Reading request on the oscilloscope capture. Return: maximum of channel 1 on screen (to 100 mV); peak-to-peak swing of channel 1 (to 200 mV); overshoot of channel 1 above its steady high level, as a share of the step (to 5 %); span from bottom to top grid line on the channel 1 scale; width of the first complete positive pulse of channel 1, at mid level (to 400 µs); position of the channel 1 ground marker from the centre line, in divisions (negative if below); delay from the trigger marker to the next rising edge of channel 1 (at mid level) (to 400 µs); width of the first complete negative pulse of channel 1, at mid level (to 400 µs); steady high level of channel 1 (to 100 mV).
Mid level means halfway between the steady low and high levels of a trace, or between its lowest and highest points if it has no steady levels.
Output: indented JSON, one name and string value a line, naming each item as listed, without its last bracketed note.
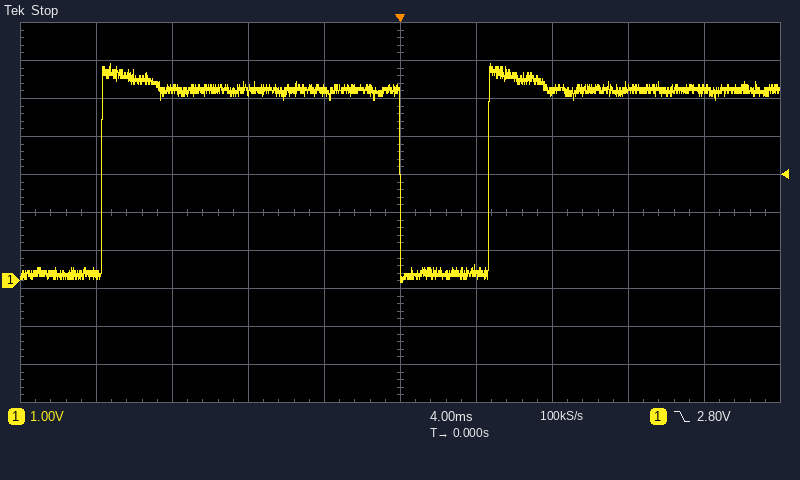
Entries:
{
  "maximum of channel 1 on screen": "5.7 V",
  "peak-to-peak swing of channel 1": "5.8 V",
  "overshoot of channel 1 above its steady high level, as a share of the step": "15 %",
  "span from bottom to top grid line on the channel 1 scale": "10 V",
  "width of the first complete positive pulse of channel 1, at mid level": "15.6 ms",
  "position of the channel 1 ground marker from the centre line, in divisions": "-1.8 div",
  "delay from the trigger marker to the next rising edge of channel 1 (at mid level)": "4.8 ms",
  "width of the first complete negative pulse of channel 1, at mid level": "4.8 ms",
  "steady high level of channel 1": "5.0 V"
}
